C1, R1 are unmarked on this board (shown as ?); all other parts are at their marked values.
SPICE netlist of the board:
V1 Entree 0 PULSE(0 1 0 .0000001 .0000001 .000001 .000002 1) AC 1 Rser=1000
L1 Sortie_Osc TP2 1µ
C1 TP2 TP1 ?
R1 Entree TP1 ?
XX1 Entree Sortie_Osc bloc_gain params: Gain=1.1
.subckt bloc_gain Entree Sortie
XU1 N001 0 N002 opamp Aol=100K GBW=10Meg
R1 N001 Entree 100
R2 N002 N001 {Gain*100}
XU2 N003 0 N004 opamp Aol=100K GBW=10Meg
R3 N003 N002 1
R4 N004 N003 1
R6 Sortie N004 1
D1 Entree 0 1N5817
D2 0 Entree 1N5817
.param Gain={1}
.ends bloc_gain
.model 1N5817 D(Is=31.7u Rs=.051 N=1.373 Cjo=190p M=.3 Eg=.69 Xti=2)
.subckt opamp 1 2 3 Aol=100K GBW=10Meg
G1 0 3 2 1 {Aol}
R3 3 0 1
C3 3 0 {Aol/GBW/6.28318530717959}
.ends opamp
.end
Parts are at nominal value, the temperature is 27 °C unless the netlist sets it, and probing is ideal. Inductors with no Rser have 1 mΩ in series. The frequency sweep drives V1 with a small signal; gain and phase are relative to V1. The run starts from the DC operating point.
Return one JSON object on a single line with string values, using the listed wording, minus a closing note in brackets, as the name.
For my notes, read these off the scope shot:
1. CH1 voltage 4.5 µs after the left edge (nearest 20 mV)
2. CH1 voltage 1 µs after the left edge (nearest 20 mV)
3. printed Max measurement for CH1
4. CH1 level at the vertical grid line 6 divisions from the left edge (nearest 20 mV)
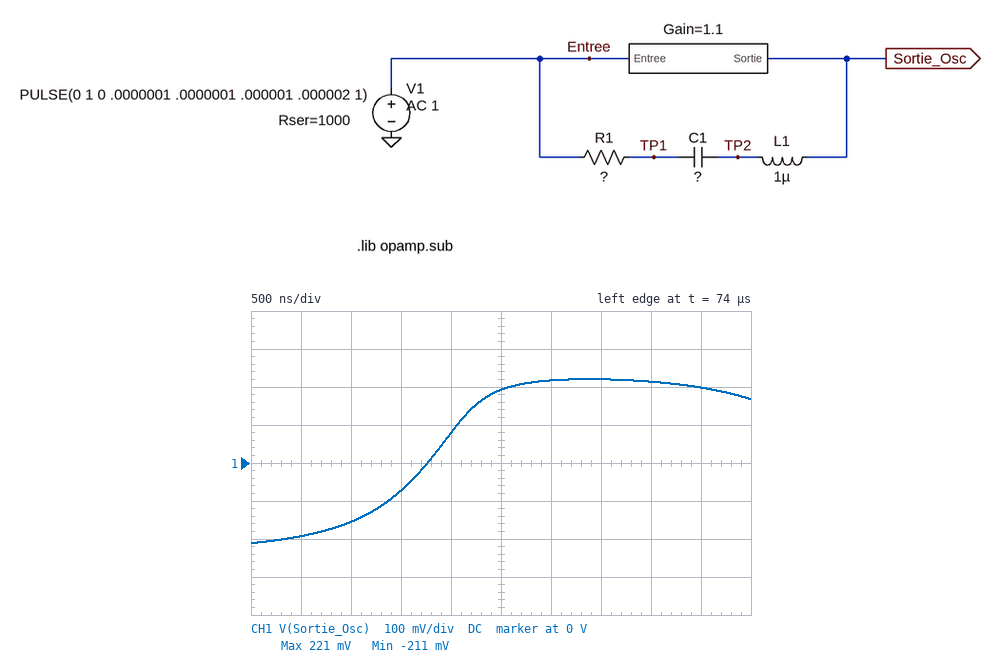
{"CH1 voltage 4.5 µs after the left edge": "200 mV", "CH1 voltage 1 µs after the left edge": "-160 mV", "printed Max measurement for CH1": "221 mV", "CH1 level at the vertical grid line 6 divisions from the left edge": "220 mV"}
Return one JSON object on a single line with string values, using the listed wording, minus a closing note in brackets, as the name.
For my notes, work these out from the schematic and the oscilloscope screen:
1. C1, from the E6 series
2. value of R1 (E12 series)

{"C1, from the E6 series": "680 nF", "value of R1": "0.68 Ω"}
